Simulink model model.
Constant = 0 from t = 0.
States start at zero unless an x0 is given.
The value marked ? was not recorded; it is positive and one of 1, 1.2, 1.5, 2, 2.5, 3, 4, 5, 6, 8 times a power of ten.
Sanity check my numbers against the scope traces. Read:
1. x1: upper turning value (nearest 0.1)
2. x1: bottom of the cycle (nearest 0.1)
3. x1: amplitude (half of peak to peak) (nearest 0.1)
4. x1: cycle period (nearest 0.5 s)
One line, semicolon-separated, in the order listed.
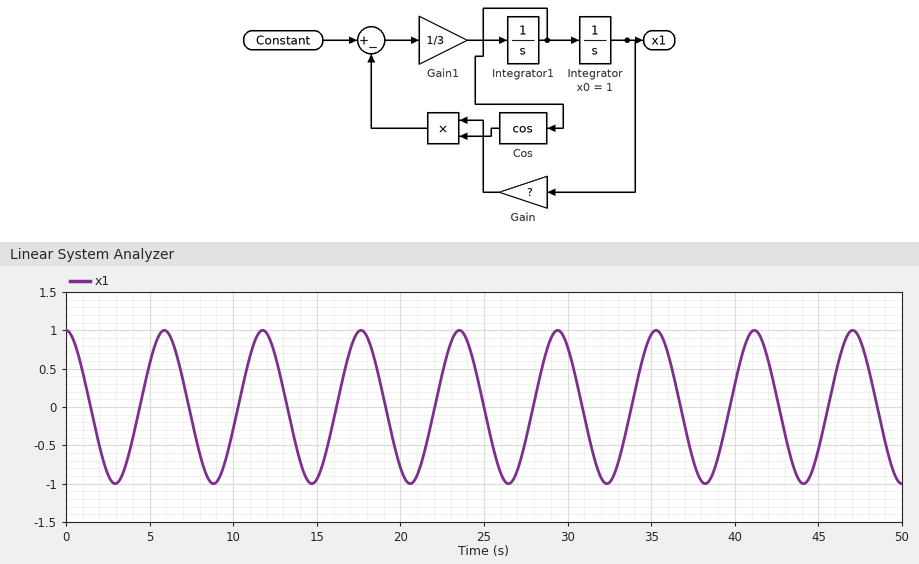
1.0; -1.0; 1.0; 6.0 s
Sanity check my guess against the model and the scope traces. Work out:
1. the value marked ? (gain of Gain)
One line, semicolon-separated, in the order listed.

4
